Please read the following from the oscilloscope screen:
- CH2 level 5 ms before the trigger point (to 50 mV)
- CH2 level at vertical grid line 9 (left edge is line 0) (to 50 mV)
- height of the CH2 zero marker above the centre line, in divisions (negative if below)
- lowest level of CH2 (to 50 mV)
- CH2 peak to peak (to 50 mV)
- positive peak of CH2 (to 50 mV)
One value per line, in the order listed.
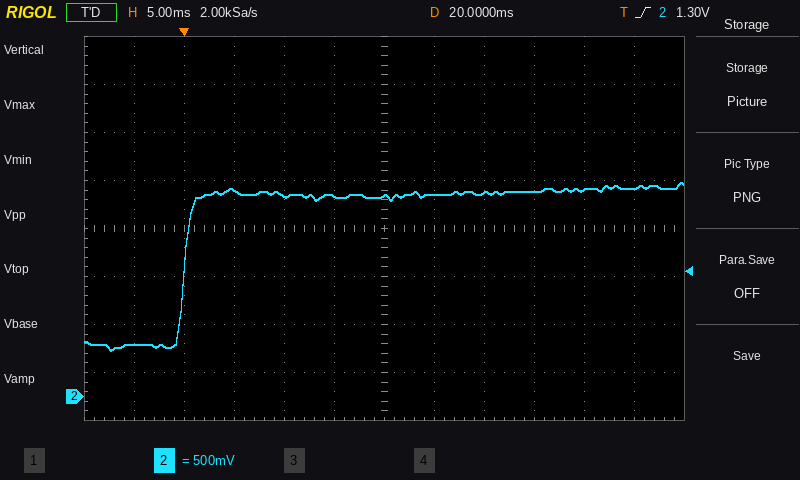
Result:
550 mV
2.15 V
-3.5 div
500 mV
1.75 V
2.25 V
